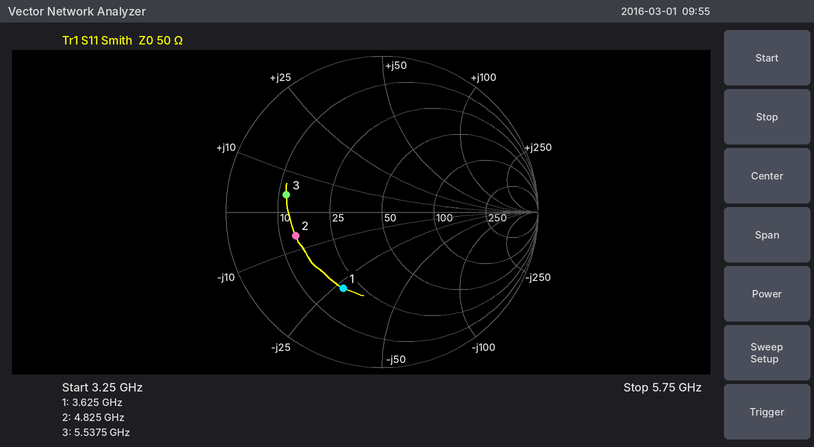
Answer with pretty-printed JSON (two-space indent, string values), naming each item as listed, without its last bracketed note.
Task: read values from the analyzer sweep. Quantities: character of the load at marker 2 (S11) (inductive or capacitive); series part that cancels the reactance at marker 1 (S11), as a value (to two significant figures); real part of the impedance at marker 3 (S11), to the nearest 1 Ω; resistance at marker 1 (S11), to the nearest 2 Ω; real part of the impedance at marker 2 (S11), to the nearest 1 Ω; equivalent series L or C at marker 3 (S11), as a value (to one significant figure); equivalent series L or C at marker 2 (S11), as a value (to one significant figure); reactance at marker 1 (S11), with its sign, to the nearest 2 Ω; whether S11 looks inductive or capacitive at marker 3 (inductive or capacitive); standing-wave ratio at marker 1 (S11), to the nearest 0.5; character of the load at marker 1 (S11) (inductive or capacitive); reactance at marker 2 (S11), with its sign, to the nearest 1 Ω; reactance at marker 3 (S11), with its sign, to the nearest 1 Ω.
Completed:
{
  "character of the load at marker 2 (S11)": "capacitive",
  "series part that cancels the reactance at marker 1 (S11), as a value": "1.2 nH",
  "real part of the impedance at marker 3 (S11), to the nearest 1 Ω": "12 Ω",
  "resistance at marker 1 (S11), to the nearest 2 Ω": "20 Ω",
  "real part of the impedance at marker 2 (S11), to the nearest 1 Ω": "14 Ω",
  "equivalent series L or C at marker 3 (S11), as a value": "100 pH",
  "equivalent series L or C at marker 2 (S11), as a value": "5 pF",
  "reactance at marker 1 (S11), with its sign, to the nearest 2 Ω": "-28 Ω",
  "whether S11 looks inductive or capacitive at marker 3": "inductive",
  "standing-wave ratio at marker 1 (S11), to the nearest 0.5": "3.5",
  "character of the load at marker 1 (S11)": "capacitive",
  "reactance at marker 2 (S11), with its sign, to the nearest 1 Ω": "-6 Ω",
  "reactance at marker 3 (S11), with its sign, to the nearest 1 Ω": "+4 Ω"
}
